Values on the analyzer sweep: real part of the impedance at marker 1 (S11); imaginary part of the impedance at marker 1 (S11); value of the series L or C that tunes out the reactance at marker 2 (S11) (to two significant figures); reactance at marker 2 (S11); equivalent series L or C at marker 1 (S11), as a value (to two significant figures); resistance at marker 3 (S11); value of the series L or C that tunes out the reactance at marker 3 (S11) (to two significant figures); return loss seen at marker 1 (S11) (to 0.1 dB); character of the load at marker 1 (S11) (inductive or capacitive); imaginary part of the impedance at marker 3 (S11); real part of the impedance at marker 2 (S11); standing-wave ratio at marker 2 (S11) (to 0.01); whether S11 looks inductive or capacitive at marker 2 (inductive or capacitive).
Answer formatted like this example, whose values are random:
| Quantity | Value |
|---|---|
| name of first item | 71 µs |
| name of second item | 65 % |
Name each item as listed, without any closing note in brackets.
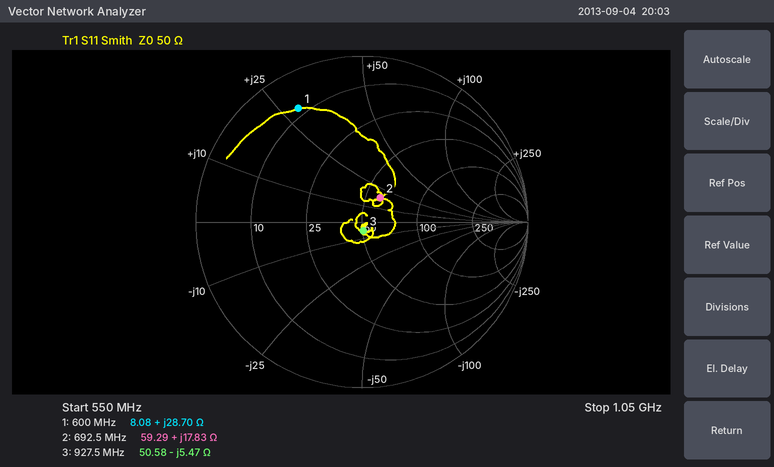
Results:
| Quantity | Value |
|---|---|
| real part of the impedance at marker 1 | 8.08 Ω |
| imaginary part of the impedance at marker 1 | +28.70 Ω |
| value of the series L or C that tunes out the reactance at marker 2 (S11) | 13 pF |
| reactance at marker 2 | +17.83 Ω |
| equivalent series L or C at marker 1 (S11), as a value | 7.6 nH |
| resistance at marker 3 | 50.58 Ω |
| value of the series L or C that tunes out the reactance at marker 3 (S11) | 940 pH |
| return loss seen at marker 1 (S11) | 2.1 dB |
| character of the load at marker 1 (S11) | inductive |
| imaginary part of the impedance at marker 3 | -5.47 Ω |
| real part of the impedance at marker 2 | 59.29 Ω |
| standing-wave ratio at marker 2 (S11) | 1.44 |
| whether S11 looks inductive or capacitive at marker 2 | inductive |
